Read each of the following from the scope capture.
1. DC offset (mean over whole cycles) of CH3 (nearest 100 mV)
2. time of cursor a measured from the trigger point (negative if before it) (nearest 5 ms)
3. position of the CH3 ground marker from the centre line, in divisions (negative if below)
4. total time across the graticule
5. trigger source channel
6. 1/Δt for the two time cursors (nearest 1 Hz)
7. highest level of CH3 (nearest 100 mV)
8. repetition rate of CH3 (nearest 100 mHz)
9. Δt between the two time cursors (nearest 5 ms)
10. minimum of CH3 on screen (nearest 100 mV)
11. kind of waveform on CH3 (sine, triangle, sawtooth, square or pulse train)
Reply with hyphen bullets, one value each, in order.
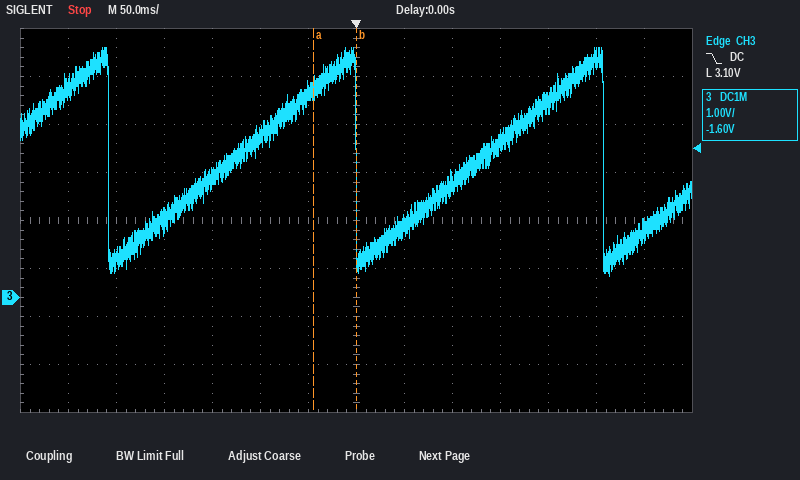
- 2.9 V
- -45 ms
- -1.6 div
- 700 ms
- CH3
- 22 Hz
- 5.2 V
- 3.9 Hz
- 45 ms
- 500 mV
- sawtooth
